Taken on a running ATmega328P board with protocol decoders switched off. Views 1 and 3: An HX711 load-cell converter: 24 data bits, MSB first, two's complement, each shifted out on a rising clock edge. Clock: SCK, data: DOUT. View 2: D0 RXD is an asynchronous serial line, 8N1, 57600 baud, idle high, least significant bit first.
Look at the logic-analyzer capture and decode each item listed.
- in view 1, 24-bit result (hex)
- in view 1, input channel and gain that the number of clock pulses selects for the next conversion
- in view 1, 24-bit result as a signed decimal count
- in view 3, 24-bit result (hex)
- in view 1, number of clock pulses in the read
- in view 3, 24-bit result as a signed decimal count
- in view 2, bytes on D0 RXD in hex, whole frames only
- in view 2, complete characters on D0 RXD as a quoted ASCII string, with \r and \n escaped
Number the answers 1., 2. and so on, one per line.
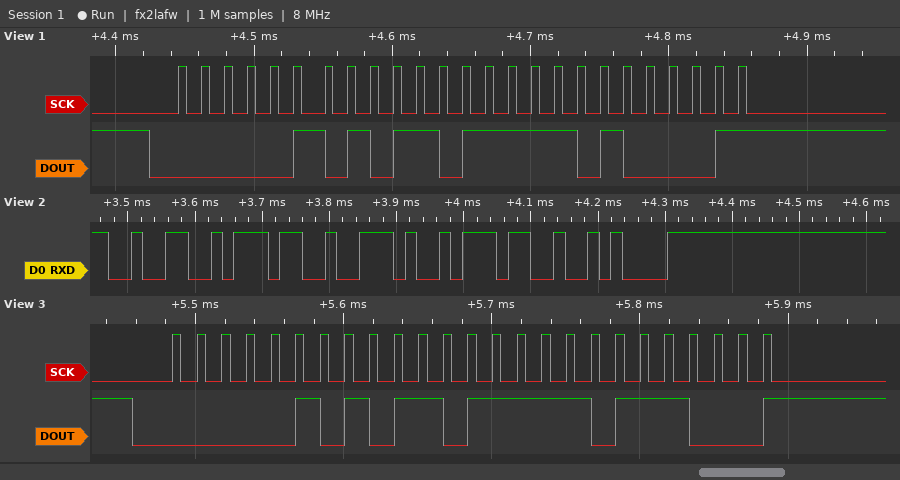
1. 0x056FA1
2. channel A, gain 128
3. 356257
4. 0x056FB8
5. 25
6. 356280
7. 32 37 2E 37 0A
8. "27.7\n"
